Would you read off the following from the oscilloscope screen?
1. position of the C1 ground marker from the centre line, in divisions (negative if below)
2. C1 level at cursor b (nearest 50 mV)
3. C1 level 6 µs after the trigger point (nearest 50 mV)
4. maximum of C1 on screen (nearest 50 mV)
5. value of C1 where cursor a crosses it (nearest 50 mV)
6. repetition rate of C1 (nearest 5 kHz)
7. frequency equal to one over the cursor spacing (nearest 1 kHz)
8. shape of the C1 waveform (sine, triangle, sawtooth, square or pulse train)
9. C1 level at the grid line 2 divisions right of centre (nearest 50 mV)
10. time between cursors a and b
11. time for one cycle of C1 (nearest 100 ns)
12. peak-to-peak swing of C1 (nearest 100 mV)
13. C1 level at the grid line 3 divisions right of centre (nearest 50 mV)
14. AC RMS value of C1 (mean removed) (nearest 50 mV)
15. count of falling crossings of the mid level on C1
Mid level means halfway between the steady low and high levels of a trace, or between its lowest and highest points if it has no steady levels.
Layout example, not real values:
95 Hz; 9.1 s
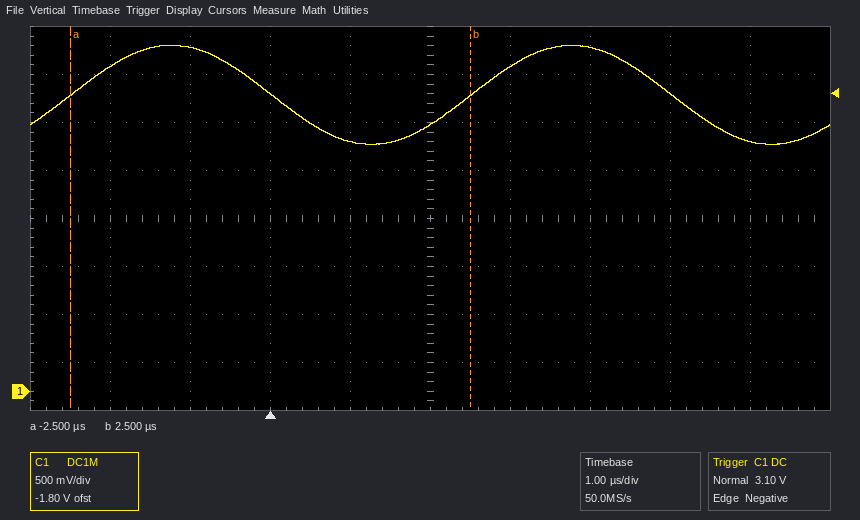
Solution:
-3.6 div; 3.10 V; 2.60 V; 3.60 V; 3.10 V; 200 kHz; 200 kHz; sine; 3.60 V; 5.0 µs; 5.0 µs; 1.00 V; 3.10 V; 350 mV; 2
